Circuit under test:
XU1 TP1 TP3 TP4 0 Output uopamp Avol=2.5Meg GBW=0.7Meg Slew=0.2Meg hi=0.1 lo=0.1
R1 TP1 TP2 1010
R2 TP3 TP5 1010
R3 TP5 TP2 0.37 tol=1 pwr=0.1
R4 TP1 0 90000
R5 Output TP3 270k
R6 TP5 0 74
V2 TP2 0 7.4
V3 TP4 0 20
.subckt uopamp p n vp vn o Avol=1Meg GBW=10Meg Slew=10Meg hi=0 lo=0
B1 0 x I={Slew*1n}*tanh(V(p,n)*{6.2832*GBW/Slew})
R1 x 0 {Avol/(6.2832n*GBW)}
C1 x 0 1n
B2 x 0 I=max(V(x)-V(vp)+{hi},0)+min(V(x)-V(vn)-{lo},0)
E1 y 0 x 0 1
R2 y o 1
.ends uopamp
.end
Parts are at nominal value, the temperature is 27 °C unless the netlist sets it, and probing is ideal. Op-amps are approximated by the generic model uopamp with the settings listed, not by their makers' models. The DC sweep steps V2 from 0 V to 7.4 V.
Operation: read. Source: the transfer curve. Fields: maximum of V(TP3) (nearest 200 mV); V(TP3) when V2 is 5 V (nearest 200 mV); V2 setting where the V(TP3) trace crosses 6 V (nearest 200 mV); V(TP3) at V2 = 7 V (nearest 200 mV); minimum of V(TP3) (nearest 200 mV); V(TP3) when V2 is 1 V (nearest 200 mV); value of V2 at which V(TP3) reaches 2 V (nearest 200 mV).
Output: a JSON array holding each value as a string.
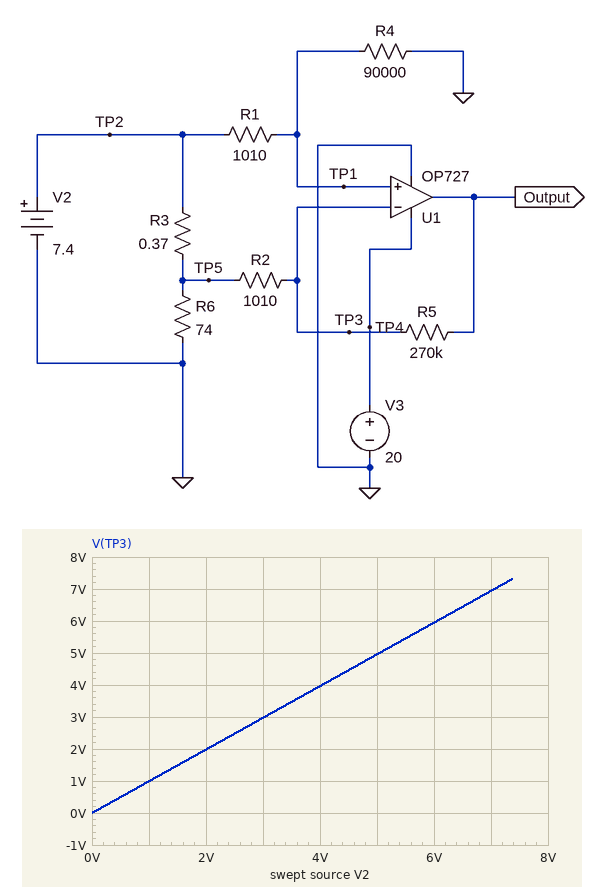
["7.4 V", "5.0 V", "6.0 V", "7.0 V", "0 V", "1.0 V", "2.0 V"]
